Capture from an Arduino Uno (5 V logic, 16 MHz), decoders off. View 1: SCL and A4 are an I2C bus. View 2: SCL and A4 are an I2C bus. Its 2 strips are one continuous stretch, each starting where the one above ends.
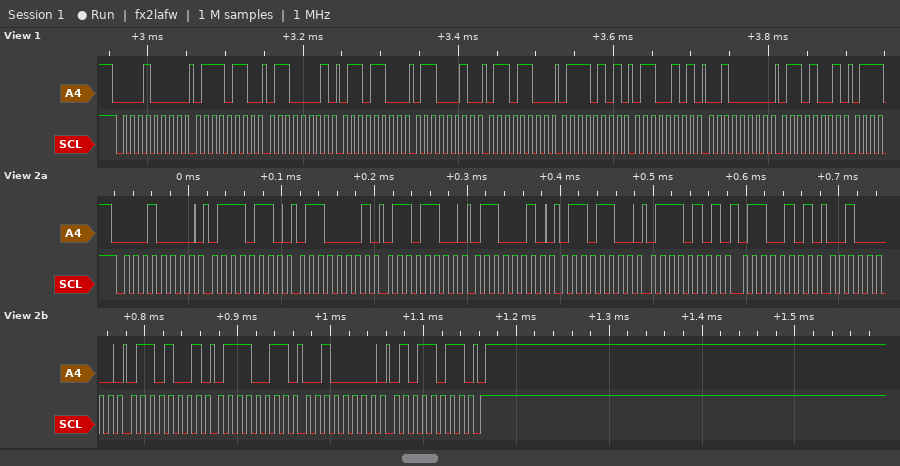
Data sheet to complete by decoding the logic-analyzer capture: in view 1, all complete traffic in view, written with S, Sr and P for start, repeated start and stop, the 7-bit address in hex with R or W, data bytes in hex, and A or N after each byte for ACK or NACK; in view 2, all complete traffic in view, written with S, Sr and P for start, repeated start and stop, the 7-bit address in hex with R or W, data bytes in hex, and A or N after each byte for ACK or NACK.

S 08W A 76 A 61 A 6C A 62 A 6C A 75 A 65 A 20 A 69 A
S 08W A 76 A 61 A 6C A 62 A 6C A 75 A 65 A 20 A 69 A 73 A 20 A 5B A P
